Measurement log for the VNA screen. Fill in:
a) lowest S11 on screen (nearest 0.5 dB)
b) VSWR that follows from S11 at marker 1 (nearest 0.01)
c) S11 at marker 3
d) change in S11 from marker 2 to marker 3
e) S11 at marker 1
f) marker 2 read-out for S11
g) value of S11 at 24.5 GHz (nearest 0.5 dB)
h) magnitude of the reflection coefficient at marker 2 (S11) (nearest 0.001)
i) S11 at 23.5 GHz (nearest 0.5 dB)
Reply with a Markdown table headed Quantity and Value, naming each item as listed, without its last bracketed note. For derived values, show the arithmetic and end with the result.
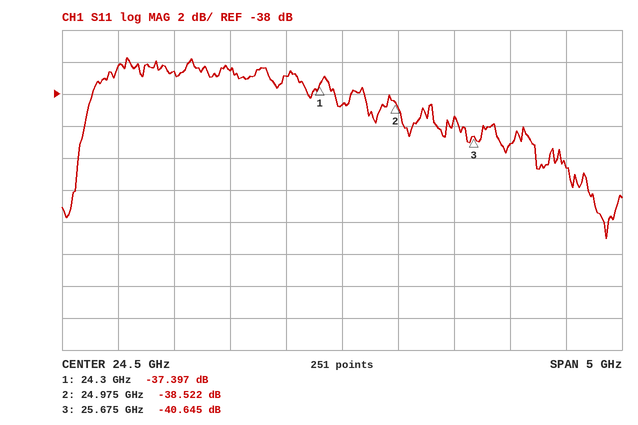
| Quantity | Value |
|---|---|
| lowest S11 on screen | -47.0 dB |
| VSWR that follows from S11 at marker 1 | (1 + 0.0135)/(1 − 0.0135) ≈ 1.03 |
| S11 at marker 3 | -40.645 dB |
| change in S11 from marker 2 to marker 3 | -40.645 − (-38.522) = -2.123 dB |
| S11 at marker 1 | -37.397 dB |
| marker 2 read-out for S11 | -38.522 dB |
| value of S11 at 24.5 GHz | -38.5 dB |
| magnitude of the reflection coefficient at marker 2 (S11) | 10^(-38.522/20) ≈ 0.012 |
| S11 at 23.5 GHz | -36.5 dB |
